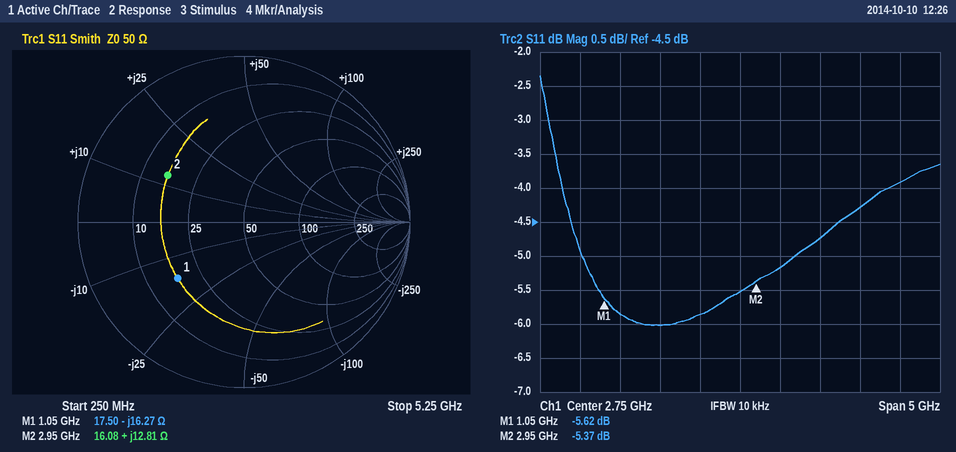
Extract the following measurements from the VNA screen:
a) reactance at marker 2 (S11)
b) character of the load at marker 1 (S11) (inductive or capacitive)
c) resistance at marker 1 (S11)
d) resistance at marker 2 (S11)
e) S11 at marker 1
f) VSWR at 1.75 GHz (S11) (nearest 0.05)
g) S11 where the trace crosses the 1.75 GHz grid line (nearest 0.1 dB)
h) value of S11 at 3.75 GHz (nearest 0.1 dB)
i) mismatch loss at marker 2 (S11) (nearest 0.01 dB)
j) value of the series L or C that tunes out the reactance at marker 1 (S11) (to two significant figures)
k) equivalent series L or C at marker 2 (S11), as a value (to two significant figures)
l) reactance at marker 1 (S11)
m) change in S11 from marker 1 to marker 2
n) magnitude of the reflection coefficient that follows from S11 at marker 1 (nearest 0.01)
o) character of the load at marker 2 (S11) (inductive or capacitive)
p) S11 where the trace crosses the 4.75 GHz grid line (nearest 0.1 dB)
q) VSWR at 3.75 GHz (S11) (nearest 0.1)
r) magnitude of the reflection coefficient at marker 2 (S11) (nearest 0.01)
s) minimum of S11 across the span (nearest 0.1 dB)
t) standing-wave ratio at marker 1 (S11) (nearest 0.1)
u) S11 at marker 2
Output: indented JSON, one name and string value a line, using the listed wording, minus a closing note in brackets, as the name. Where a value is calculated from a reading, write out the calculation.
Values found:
{
  "reactance at marker 2": "+12.81 Ω",
  "character of the load at marker 1 (S11)": "capacitive",
  "resistance at marker 1": "17.50 Ω",
  "resistance at marker 2": "16.08 Ω",
  "S11 at marker 1": "-5.62 dB",
  "VSWR at 1.75 GHz (S11)": "|Γ| = 10^(-6/20) = 0.5012; VSWR = (1 + 0.5012)/(1 − 0.5012) ≈ 3.01, so 3.00 to the nearest 0.05",
  "S11 where the trace crosses the 1.75 GHz grid line": "-6.0 dB",
  "value of S11 at 3.75 GHz": "-4.7 dB",
  "mismatch loss at marker 2 (S11)": "−10 log10(1 − 10^(-5.37/10)) ≈ 1.49 dB",
  "value of the series L or C that tunes out the reactance at marker 1 (S11)": "L = 16.27 Ω/(2π × 1.05 GHz) ≈ 2.5 nH",
  "equivalent series L or C at marker 2 (S11), as a value": "L = 12.81 Ω/(2π × 2.95 GHz) ≈ 691 pH, so 690 pH to two significant figures",
  "reactance at marker 1": "-16.27 Ω",
  "change in S11 from marker 1 to marker 2": "-5.37 − (-5.62) = 0.25 dB",
  "magnitude of the reflection coefficient that follows from S11 at marker 1": "10^(-5.62/20) ≈ 0.52",
  "character of the load at marker 2 (S11)": "inductive",
  "S11 where the trace crosses the 4.75 GHz grid line": "-3.9 dB",
  "VSWR at 3.75 GHz (S11)": "|Γ| = 10^(-4.7/20) = 0.5821; VSWR = (1 + 0.5821)/(1 − 0.5821) ≈ 3.8",
  "magnitude of the reflection coefficient at marker 2 (S11)": "0.54",
  "minimum of S11 across the span": "-6.0 dB",
  "standing-wave ratio at marker 1 (S11)": "3.2",
  "S11 at marker 2": "-5.37 dB"
}
